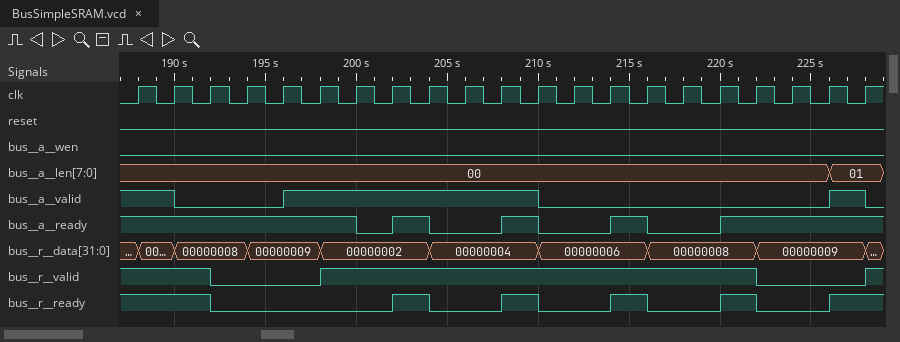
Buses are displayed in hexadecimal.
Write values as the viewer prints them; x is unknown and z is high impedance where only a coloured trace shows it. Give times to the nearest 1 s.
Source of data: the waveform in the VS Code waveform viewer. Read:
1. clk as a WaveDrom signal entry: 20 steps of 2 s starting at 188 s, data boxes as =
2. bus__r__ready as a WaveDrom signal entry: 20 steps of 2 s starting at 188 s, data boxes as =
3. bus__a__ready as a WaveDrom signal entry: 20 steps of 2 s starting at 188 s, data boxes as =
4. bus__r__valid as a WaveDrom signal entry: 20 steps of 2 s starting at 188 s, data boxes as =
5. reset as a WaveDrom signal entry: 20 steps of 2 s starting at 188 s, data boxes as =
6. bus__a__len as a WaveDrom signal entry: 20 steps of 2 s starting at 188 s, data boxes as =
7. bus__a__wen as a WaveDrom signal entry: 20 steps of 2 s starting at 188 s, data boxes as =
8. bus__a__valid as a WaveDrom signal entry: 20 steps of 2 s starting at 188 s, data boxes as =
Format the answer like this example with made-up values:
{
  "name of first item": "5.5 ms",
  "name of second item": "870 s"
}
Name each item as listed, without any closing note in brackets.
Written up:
{
  "clk as a WaveDrom signal entry: 20 steps of 2 s starting at 188 s, data boxes as =": "{name: 'clk', wave: 'p...................'}",
  "bus__r__ready as a WaveDrom signal entry: 20 steps of 2 s starting at 188 s, data boxes as =": "{name: 'bus__r__ready', wave: '1.0....10.10.10.10.1'}",
  "bus__a__ready as a WaveDrom signal entry: 20 steps of 2 s starting at 188 s, data boxes as =": "{name: 'bus__a__ready', wave: '1.....010.10.10.1...'}",
  "bus__r__valid as a WaveDrom signal entry: 20 steps of 2 s starting at 188 s, data boxes as =": "{name: 'bus__r__valid', wave: '1.0..1...........0..'}",
  "reset as a WaveDrom signal entry: 20 steps of 2 s starting at 188 s, data boxes as =": "{name: 'reset', wave: '0...................'}",
  "bus__a__len as a WaveDrom signal entry: 20 steps of 2 s starting at 188 s, data boxes as =": "{name: 'bus__a__len', wave: '=..................=', data: '00 01'}",
  "bus__a__wen as a WaveDrom signal entry: 20 steps of 2 s starting at 188 s, data boxes as =": "{name: 'bus__a__wen', wave: '0...................'}",
  "bus__a__valid as a WaveDrom signal entry: 20 steps of 2 s starting at 188 s, data boxes as =": "{name: 'bus__a__valid', wave: '10..1......0.......1'}"
}
